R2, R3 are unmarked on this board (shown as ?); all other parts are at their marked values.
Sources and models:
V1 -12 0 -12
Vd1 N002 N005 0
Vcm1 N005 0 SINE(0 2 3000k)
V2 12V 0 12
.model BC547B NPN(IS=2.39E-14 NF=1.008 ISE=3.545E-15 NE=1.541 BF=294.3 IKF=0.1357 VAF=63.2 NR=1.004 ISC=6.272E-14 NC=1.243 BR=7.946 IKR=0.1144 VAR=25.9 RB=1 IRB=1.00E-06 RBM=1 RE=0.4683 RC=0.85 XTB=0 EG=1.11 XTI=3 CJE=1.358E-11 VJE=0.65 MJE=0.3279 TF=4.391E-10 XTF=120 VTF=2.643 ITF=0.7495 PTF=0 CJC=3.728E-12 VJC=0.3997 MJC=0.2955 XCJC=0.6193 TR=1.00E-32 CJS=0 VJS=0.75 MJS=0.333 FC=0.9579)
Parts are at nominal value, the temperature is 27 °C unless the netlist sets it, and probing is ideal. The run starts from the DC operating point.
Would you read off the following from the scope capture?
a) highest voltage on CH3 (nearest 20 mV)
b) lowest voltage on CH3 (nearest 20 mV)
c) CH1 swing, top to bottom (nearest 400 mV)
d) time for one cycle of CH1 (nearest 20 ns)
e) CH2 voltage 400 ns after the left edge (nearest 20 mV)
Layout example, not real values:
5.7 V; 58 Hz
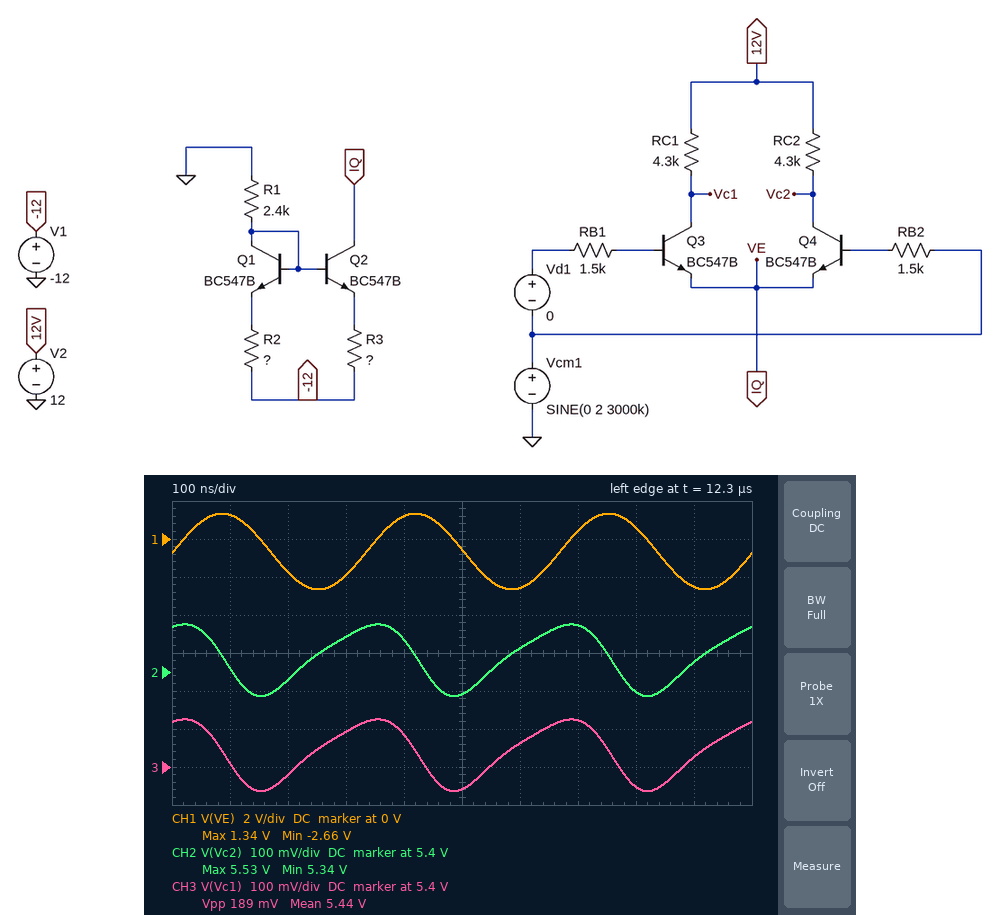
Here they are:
5.52 V; 5.34 V; 4.0 V; 340 ns; 5.48 V
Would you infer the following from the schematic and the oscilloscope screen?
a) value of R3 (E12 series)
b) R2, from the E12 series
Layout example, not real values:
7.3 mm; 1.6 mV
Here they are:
180 Ω; 120 Ω
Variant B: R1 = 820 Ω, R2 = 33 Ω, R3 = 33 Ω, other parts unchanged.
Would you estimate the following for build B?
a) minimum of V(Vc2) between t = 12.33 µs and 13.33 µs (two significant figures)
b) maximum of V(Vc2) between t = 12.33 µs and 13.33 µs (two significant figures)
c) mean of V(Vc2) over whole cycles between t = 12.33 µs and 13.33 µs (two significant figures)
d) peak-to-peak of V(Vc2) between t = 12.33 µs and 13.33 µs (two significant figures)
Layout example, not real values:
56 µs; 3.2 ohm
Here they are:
-6.2 V; -3.3 V; -4.8 V; 2.9 V
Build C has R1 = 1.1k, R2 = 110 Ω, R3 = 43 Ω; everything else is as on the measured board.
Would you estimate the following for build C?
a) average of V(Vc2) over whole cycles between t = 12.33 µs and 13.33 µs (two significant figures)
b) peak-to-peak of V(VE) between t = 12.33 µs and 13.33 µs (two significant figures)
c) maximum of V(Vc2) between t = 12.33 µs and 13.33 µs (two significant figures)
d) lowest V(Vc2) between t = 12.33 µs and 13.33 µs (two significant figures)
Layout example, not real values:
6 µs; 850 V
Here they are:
-10 V; 2.3 V; -8.7 V; -11 V
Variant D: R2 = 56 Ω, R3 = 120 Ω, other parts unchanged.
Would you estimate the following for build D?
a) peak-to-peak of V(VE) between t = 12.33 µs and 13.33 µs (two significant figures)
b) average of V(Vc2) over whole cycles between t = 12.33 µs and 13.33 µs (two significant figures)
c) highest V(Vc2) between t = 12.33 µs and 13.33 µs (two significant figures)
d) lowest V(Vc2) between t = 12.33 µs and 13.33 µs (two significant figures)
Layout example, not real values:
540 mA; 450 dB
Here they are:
4.0 V; 7.0 V; 7.1 V; 6.9 V
